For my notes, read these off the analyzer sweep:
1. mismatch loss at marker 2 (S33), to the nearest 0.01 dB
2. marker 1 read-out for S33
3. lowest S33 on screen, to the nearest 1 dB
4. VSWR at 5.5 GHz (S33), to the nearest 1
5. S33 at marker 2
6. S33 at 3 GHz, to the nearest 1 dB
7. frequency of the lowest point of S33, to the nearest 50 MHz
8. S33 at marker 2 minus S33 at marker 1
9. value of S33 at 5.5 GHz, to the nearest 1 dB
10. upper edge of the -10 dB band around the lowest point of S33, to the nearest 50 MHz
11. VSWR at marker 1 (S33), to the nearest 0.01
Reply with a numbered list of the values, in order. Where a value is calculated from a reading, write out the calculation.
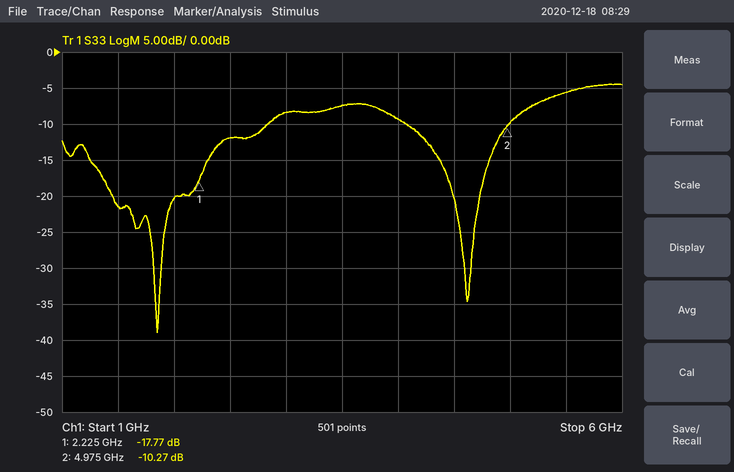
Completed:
1. −10 log10(1 − 10^(-10.27/10)) ≈ 0.43 dB
2. -17.77 dB
3. -39 dB
4. |Γ| = 10^(-6/20) = 0.5012; VSWR = (1 + 0.5012)/(1 − 0.5012) ≈ 3
5. -10.27 dB
6. -8 dB
7. 1.85 GHz
8. -10.27 − (-17.77) = 7.50 dB
9. -6 dB
10. 2.85 GHz
11. (1 + 0.1293)/(1 − 0.1293) ≈ 1.30
